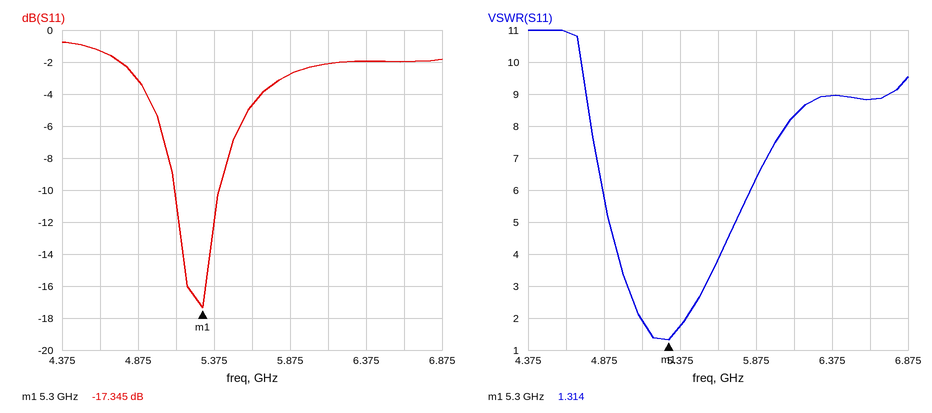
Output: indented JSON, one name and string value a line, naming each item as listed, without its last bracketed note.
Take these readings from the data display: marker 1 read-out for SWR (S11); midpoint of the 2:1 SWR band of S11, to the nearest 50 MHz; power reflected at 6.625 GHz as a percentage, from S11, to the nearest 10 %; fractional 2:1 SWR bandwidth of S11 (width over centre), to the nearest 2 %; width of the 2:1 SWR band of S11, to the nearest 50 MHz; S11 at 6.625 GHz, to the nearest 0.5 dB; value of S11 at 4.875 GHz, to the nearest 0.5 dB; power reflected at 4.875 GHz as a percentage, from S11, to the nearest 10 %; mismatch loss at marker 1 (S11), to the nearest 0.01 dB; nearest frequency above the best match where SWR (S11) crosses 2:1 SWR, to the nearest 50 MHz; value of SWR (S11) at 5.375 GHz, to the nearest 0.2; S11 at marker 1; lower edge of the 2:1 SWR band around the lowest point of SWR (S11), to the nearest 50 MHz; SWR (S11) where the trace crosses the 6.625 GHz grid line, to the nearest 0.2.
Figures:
{
  "marker 1 read-out for SWR": "1.314",
  "midpoint of the 2:1 SWR band of S11, to the nearest 50 MHz": "5.25 GHz",
  "power reflected at 6.625 GHz as a percentage, from S11, to the nearest 10 %": "60 %",
  "fractional 2:1 SWR bandwidth of S11 (width over centre), to the nearest 2 %": "6 %",
  "width of the 2:1 SWR band of S11, to the nearest 50 MHz": "300 MHz",
  "S11 at 6.625 GHz, to the nearest 0.5 dB": "-2.0 dB",
  "value of S11 at 4.875 GHz, to the nearest 0.5 dB": "-3.0 dB",
  "power reflected at 4.875 GHz as a percentage, from S11, to the nearest 10 %": "50 %",
  "mismatch loss at marker 1 (S11), to the nearest 0.01 dB": "0.08 dB",
  "nearest frequency above the best match where SWR (S11) crosses 2:1 SWR, to the nearest 50 MHz": "5.40 GHz",
  "value of SWR (S11) at 5.375 GHz, to the nearest 0.2": "1.8",
  "S11 at marker 1": "-17.345 dB",
  "lower edge of the 2:1 SWR band around the lowest point of SWR (S11), to the nearest 50 MHz": "5.10 GHz",
  "SWR (S11) where the trace crosses the 6.625 GHz grid line, to the nearest 0.2": "8.8"
}
